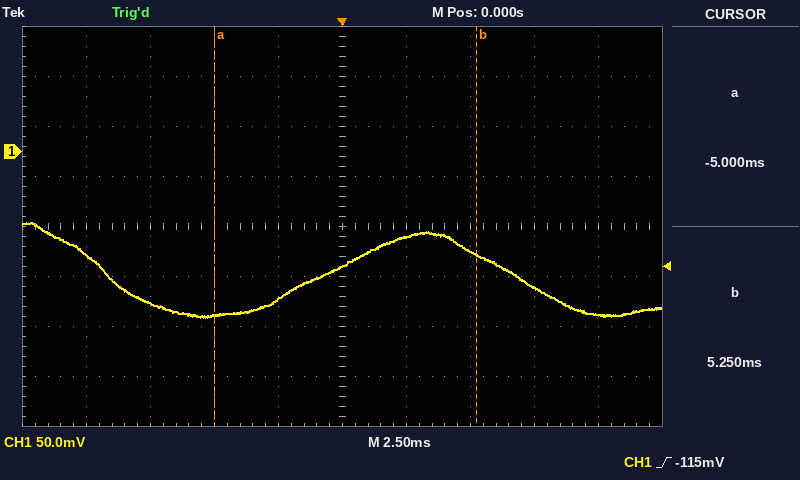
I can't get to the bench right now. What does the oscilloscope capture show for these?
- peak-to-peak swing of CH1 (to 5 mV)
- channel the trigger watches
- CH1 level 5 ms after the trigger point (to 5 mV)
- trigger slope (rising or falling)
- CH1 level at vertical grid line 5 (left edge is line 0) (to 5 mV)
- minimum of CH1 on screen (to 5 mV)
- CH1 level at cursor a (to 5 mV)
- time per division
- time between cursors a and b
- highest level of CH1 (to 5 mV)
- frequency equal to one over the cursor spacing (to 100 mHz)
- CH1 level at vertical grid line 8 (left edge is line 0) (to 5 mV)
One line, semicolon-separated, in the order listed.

95 mV; CH1; -100 mV; rising; -115 mV; -165 mV; -165 mV; 2.5 ms; 10.25 ms; -70 mV; 97.6 Hz; -135 mV
